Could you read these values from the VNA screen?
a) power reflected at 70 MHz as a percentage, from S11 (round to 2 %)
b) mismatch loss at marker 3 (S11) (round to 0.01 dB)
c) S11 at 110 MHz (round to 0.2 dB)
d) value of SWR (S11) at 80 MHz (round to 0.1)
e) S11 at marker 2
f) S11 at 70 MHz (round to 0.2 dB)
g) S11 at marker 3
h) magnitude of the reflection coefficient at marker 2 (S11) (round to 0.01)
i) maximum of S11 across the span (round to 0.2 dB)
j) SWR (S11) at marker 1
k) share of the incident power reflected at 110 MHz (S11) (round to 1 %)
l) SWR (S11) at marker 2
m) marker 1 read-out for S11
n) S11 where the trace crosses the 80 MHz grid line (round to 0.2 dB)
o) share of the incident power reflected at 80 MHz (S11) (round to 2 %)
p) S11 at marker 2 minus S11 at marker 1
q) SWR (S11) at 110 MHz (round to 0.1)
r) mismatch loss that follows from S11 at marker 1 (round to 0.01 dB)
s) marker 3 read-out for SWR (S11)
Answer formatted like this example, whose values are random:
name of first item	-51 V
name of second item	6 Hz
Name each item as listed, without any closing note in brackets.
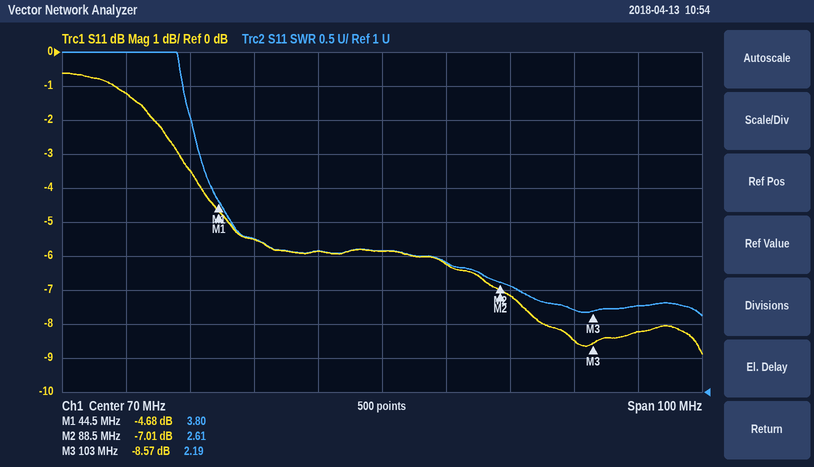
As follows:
power reflected at 70 MHz as a percentage, from S11	26 %
mismatch loss at marker 3 (S11)	0.65 dB
S11 at 110 MHz	-8.2 dB
value of SWR (S11) at 80 MHz	2.9
S11 at marker 2	-7.01 dB
S11 at 70 MHz	-5.8 dB
S11 at marker 3	-8.57 dB
magnitude of the reflection coefficient at marker 2 (S11)	0.45
maximum of S11 across the span	-0.6 dB
SWR (S11) at marker 1	3.80
share of the incident power reflected at 110 MHz (S11)	15 %
SWR (S11) at marker 2	2.61
marker 1 read-out for S11	-4.68 dB
S11 where the trace crosses the 80 MHz grid line	-6.2 dB
share of the incident power reflected at 80 MHz (S11)	24 %
S11 at marker 2 minus S11 at marker 1	-2.33 dB
SWR (S11) at 110 MHz	2.3
mismatch loss that follows from S11 at marker 1	1.81 dB
marker 3 read-out for SWR	2.19
